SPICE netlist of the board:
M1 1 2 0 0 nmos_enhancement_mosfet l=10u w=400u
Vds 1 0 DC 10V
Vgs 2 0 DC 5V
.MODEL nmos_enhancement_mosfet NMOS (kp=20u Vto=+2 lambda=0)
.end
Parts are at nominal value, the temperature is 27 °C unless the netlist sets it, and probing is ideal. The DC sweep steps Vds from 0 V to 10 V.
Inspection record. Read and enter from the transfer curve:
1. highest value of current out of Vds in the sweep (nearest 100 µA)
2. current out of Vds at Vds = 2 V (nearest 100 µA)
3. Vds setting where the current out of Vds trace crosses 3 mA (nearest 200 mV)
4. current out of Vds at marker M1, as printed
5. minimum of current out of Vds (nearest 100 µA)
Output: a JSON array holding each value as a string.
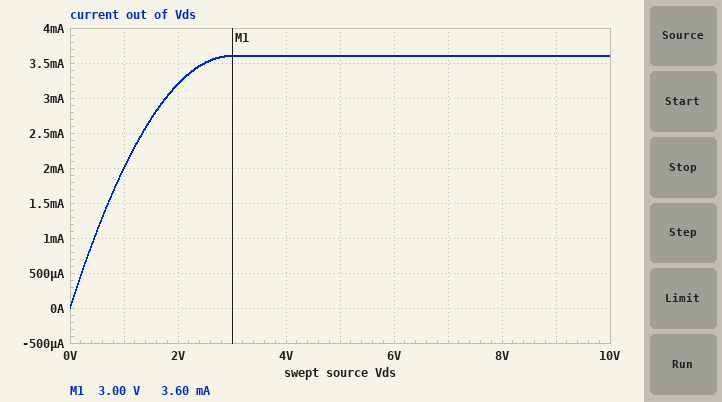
["3.6 mA", "3.2 mA", "1.8 V", "3.60 mA", "0 A"]
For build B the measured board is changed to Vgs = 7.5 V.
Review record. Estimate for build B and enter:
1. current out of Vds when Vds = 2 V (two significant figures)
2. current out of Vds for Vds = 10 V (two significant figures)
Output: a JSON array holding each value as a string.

["7.2 mA", "12 mA"]
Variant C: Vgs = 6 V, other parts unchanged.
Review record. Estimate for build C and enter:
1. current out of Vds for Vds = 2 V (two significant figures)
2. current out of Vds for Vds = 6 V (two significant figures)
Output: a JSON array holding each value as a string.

["4.8 mA", "6.4 mA"]
